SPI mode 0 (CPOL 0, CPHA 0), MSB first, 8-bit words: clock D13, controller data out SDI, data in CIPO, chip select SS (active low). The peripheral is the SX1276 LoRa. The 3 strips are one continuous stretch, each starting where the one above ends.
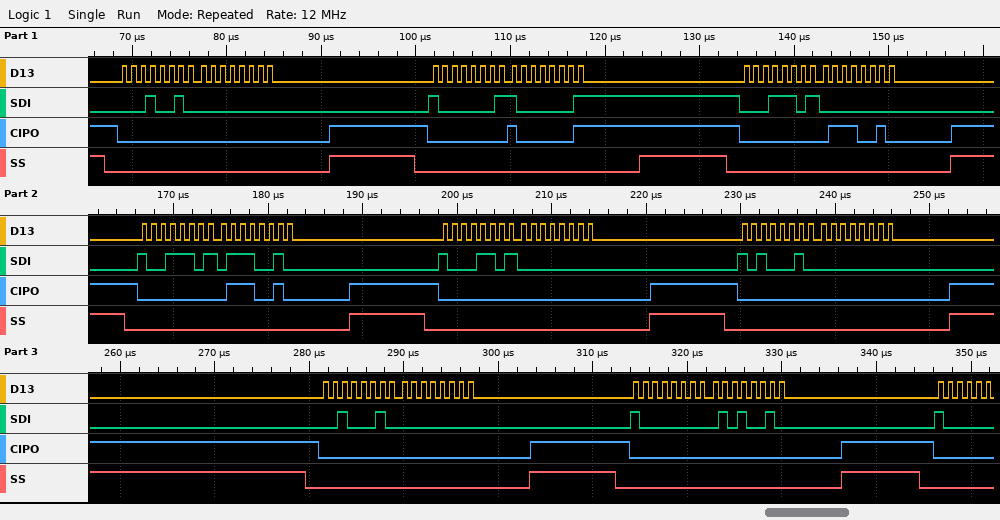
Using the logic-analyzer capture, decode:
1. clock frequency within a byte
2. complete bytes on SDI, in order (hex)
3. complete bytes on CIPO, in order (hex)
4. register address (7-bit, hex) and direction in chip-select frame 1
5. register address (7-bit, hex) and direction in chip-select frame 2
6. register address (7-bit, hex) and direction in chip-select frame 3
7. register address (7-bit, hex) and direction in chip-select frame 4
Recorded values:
1 MHz
12 00 81 81 1D 00 9D 72 8D 00 A2 00 22 00 80 52
00 00 00 81 00 72 00 72 00 00 00 00 00 00 00 00
0x12 read
0x01 write
0x1D read
0x1D write
